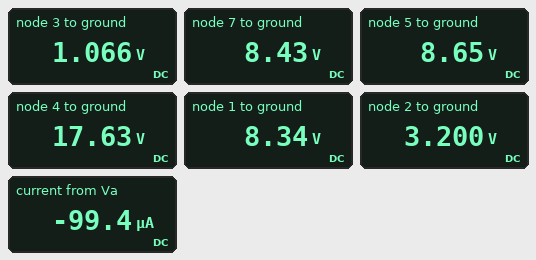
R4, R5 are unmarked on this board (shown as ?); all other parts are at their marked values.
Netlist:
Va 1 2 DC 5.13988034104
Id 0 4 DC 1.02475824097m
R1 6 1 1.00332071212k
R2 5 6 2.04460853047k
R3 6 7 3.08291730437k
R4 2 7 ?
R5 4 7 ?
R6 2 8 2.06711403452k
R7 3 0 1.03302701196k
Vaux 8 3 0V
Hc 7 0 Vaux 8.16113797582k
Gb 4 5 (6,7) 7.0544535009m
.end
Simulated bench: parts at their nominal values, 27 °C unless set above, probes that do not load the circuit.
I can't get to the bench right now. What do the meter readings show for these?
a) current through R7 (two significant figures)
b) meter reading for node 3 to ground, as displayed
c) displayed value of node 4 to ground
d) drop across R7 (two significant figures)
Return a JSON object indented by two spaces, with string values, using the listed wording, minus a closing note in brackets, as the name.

{
  "current through R7": "1.0 mA",
  "meter reading for node 3 to ground, as displayed": "1.066 V",
  "displayed value of node 4 to ground": "17.63 V",
  "drop across R7": "1.1 V"
}
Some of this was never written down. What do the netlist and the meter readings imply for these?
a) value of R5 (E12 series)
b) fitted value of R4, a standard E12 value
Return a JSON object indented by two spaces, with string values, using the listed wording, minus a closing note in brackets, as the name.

{
  "value of R5": "10 kΩ",
  "fitted value of R4, a standard E12 value": "5.6 kΩ"
}
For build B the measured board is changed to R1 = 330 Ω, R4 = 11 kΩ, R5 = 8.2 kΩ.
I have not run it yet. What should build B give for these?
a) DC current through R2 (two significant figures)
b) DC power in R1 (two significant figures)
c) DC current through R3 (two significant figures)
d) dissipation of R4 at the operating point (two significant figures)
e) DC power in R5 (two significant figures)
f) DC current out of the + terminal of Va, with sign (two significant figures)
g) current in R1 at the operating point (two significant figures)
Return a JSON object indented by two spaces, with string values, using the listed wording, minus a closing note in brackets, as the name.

{
  "DC current through R2": "590 µA",
  "DC power in R1": "100 µW",
  "DC current through R3": "27 µA",
  "dissipation of R4 at the operating point": "2.5 mW",
  "DC power in R5": "1.6 mW",
  "DC current out of the + terminal of Va, with sign": "-560 µA",
  "current in R1 at the operating point": "560 µA"
}
